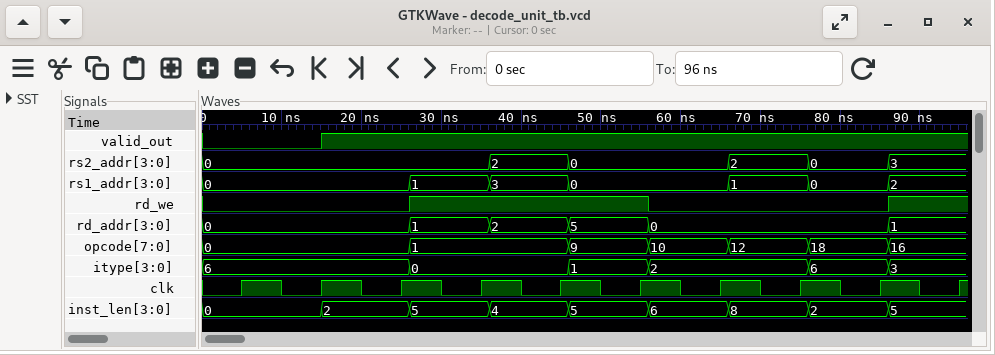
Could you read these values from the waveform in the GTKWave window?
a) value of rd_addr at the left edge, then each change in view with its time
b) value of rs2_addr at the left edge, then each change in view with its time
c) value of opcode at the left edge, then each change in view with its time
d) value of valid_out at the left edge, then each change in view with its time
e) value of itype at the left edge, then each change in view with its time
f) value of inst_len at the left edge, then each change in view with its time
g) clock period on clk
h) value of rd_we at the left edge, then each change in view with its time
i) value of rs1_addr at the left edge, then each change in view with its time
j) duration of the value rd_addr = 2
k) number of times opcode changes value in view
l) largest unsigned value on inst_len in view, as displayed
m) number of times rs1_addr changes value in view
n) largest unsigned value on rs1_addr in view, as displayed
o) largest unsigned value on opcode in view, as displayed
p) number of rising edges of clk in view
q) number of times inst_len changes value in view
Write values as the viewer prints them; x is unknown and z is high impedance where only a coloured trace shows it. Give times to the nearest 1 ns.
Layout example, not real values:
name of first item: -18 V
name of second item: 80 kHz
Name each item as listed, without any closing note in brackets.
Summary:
value of rd_addr at the left edge, then each change in view with its time: 0, 1 at 26 ns, 2 at 36 ns, 5 at 46 ns, 0 at 56 ns, 1 at 86 ns
value of rs2_addr at the left edge, then each change in view with its time: 0, 2 at 36 ns, 0 at 46 ns, 2 at 66 ns, 0 at 76 ns, 3 at 86 ns
value of opcode at the left edge, then each change in view with its time: 0, 1 at 26 ns, 9 at 46 ns, 10 at 56 ns, 12 at 66 ns, 18 at 76 ns, 16 at 86 ns
value of valid_out at the left edge, then each change in view with its time: 0, 1 at 15 ns
value of itype at the left edge, then each change in view with its time: 6, 0 at 26 ns, 1 at 46 ns, 2 at 56 ns, 6 at 76 ns, 3 at 86 ns
value of inst_len at the left edge, then each change in view with its time: 0, 2 at 15 ns, 5 at 26 ns, 4 at 36 ns, 5 at 46 ns, 6 at 56 ns, 8 at 66 ns, 2 at 76 ns, 5 at 86 ns
clock period on clk: 10 ns
value of rd_we at the left edge, then each change in view with its time: 0, 1 at 26 ns, 0 at 56 ns, 1 at 86 ns
value of rs1_addr at the left edge, then each change in view with its time: 0, 1 at 26 ns, 3 at 36 ns, 0 at 46 ns, 1 at 66 ns, 0 at 76 ns, 2 at 86 ns
duration of the value rd_addr = 2: 10 ns
number of times opcode changes value in view: 6
largest unsigned value on inst_len in view, as displayed: 8
number of times rs1_addr changes value in view: 6
largest unsigned value on rs1_addr in view, as displayed: 3
largest unsigned value on opcode in view, as displayed: 18
number of rising edges of clk in view: 10
number of times inst_len changes value in view: 8
